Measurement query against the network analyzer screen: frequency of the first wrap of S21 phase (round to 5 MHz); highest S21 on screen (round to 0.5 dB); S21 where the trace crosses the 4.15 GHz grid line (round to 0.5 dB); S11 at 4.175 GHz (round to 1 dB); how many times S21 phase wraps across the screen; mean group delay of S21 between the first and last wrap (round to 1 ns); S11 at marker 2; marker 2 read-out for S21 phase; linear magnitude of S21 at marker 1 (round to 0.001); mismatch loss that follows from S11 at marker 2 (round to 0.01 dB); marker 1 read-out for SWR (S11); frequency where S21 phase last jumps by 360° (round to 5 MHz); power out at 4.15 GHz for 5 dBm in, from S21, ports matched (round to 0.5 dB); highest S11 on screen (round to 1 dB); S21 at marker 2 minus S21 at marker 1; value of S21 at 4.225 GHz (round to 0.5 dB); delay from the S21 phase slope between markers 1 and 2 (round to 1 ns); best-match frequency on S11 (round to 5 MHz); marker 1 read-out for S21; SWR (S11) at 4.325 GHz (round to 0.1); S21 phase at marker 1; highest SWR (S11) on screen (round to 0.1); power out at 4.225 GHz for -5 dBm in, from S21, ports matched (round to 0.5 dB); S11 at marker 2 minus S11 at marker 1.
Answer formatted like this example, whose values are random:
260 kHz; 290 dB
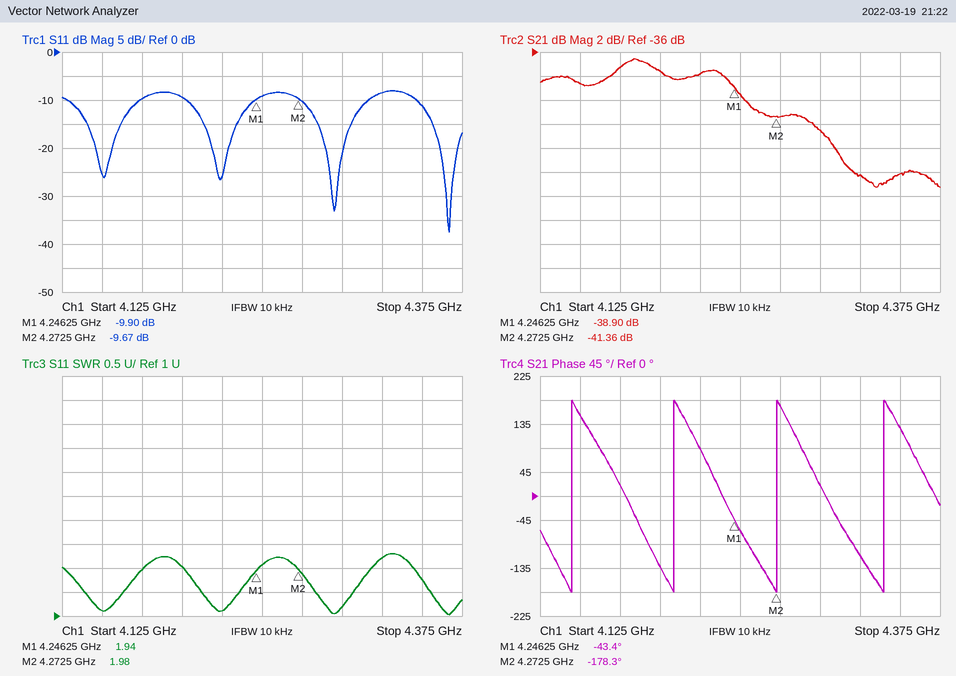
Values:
4.145 GHz; -36.5 dB; -38.5 dB; -10 dB; 4; 15 ns; -9.67 dB; -178.3°; 0.011; 0.50 dB; 1.94; 4.340 GHz; -33.5 dBm; -8 dB; -2.46 dB; -38.0 dB; 14 ns; 4.365 GHz; -38.90 dB; 2.2; -43.4°; 2.3; -43.0 dBm; 0.23 dB
